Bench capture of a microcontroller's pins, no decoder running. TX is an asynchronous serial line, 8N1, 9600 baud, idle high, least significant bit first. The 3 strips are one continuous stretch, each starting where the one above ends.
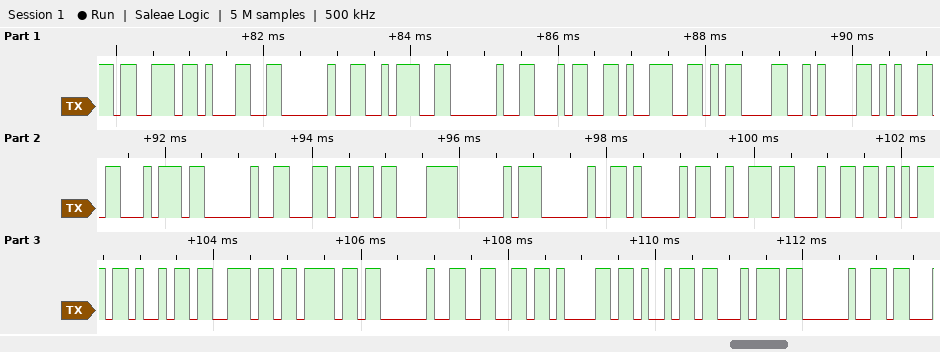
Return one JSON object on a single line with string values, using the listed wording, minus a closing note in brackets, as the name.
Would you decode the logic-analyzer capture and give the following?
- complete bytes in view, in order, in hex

{"complete bytes in view, in order, in hex": "0x73 0x31 0x20 0x3A 0x20 0x34 0x39 0x0D 0x0A 0x65 0x74 0x20 0x6C 0xC3 0xA0 0x20 0x41 0x72 0x64 0x75 0x69 0x6E 0x6F 0x20 0x66 0x61 0x69 0x74 0x20"}
